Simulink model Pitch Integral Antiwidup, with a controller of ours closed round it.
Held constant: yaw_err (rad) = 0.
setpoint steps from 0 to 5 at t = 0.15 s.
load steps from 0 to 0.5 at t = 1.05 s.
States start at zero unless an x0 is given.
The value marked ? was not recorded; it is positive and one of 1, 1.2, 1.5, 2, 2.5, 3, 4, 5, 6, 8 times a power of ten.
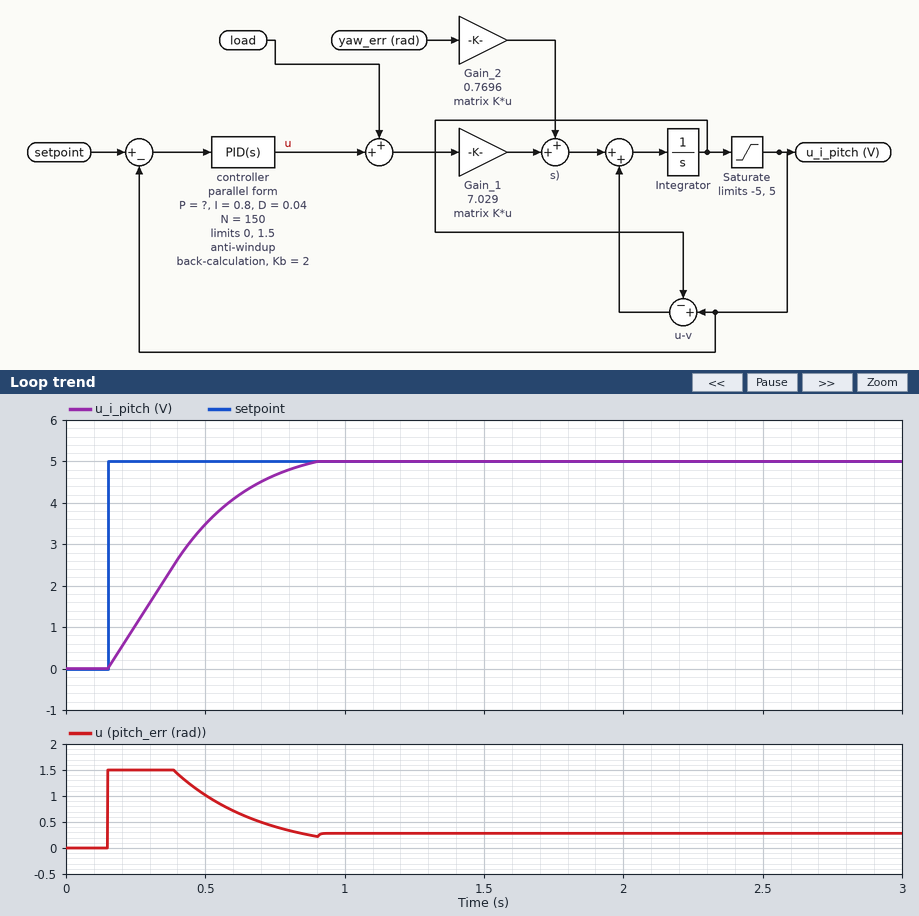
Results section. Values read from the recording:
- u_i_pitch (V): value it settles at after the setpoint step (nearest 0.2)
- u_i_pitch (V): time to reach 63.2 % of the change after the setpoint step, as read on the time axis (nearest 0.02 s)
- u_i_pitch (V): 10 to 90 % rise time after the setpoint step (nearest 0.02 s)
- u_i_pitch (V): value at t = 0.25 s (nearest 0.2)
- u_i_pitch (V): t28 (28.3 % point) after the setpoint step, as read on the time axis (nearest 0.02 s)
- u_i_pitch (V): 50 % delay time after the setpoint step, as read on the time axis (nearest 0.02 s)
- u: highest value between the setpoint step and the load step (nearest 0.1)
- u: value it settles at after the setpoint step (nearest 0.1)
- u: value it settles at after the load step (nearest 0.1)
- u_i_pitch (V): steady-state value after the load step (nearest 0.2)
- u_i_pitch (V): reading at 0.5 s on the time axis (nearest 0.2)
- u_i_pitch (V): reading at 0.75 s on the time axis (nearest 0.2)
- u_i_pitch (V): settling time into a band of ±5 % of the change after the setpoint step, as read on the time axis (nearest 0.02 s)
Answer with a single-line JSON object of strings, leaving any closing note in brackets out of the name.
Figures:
{"u_i_pitch (V): value it settles at after the setpoint step": "5.0", "u_i_pitch (V): time to reach 63.2 % of the change after the setpoint step, as read on the time axis": "0.46 s", "u_i_pitch (V): 10 to 90 % rise time after the setpoint step": "0.50 s", "u_i_pitch (V): value at t = 0.25 s": "1.0", "u_i_pitch (V): t28 (28.3 % point) after the setpoint step, as read on the time axis": "0.28 s", "u_i_pitch (V): 50 % delay time after the setpoint step, as read on the time axis": "0.38 s", "u: highest value between the setpoint step and the load step": "1.5", "u: value it settles at after the setpoint step": "0.3", "u: value it settles at after the load step": "0.3", "u_i_pitch (V): steady-state value after the load step": "5.0", "u_i_pitch (V): reading at 0.5 s on the time axis": "3.4", "u_i_pitch (V): reading at 0.75 s on the time axis": "4.6", "u_i_pitch (V): settling time into a band of ±5 % of the change after the setpoint step, as read on the time axis": "0.78 s"}
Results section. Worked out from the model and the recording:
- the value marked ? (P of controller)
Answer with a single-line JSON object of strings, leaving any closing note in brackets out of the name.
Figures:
{"the value marked ?": "0.8"}
